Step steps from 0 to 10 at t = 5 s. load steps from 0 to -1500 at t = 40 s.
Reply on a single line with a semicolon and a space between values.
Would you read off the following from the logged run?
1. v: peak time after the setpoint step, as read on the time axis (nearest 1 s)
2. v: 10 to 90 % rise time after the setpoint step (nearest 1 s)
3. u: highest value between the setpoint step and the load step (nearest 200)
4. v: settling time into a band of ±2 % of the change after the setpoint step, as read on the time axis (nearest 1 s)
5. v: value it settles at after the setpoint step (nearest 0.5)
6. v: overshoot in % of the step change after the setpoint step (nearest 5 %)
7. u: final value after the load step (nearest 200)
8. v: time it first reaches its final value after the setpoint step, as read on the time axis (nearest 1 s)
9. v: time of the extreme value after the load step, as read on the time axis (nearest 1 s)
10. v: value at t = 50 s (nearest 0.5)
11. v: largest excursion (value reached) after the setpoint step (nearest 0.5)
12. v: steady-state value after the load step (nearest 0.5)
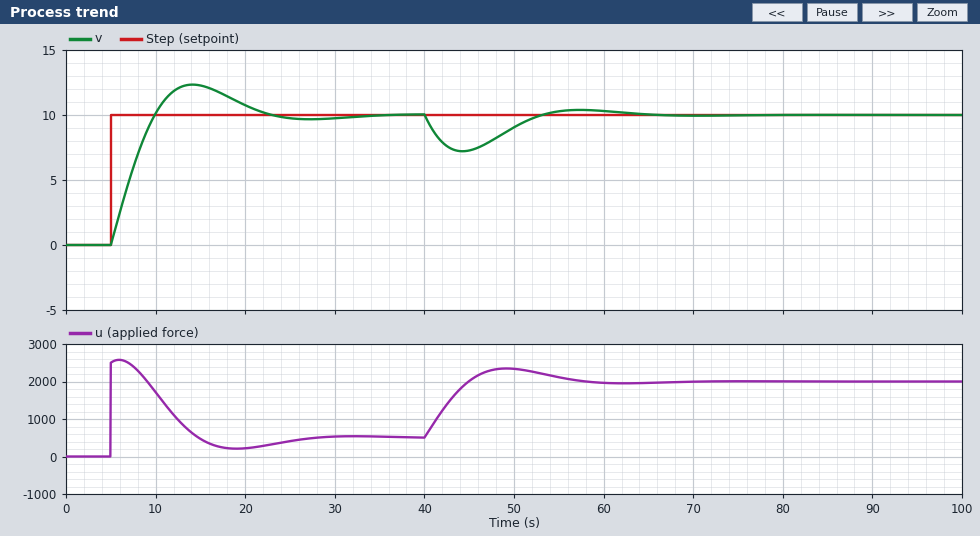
14 s; 4 s; 2600; 31 s; 10.0; 25 %; 2000; 10 s; 44 s; 9.0; 12.5; 10.0
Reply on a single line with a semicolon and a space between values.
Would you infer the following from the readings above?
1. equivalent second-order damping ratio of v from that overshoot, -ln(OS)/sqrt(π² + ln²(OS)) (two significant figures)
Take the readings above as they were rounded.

0.40
